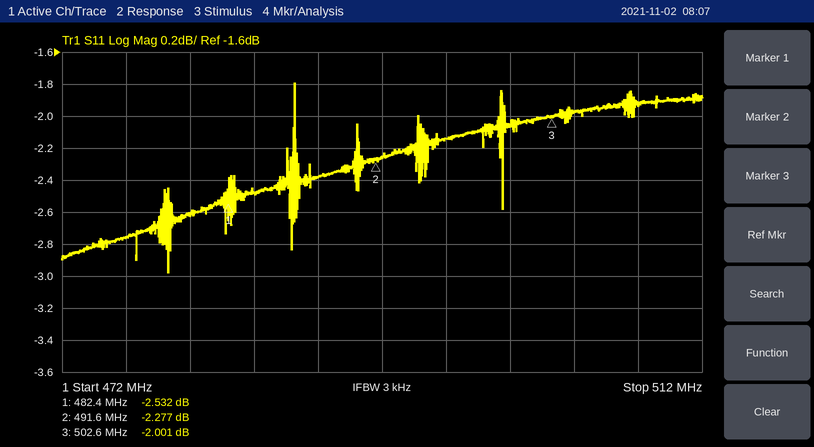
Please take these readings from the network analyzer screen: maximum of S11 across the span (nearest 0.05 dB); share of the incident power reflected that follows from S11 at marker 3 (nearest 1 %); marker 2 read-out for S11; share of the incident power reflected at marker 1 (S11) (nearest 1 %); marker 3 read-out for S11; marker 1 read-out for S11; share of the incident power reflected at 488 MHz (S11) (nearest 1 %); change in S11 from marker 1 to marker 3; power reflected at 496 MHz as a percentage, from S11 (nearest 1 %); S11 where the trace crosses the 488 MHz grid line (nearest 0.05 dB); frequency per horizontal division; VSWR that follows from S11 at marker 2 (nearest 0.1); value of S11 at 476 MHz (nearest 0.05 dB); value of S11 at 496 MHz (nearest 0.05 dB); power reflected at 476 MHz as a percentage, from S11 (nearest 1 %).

-1.80 dB
63 %
-2.277 dB
56 %
-2.001 dB
-2.532 dB
58 %
0.531 dB
61 %
-2.40 dB
4 MHz
7.7
-2.75 dB
-2.15 dB
53 %
